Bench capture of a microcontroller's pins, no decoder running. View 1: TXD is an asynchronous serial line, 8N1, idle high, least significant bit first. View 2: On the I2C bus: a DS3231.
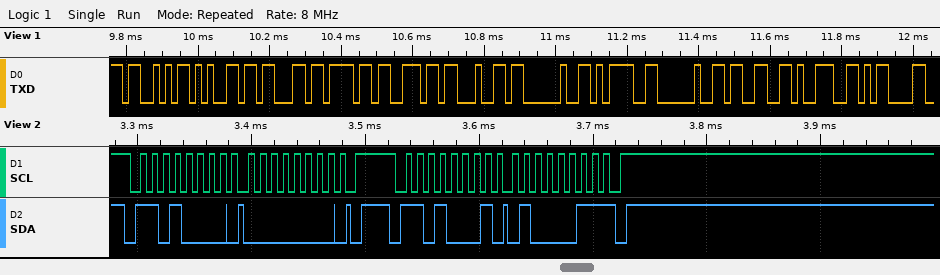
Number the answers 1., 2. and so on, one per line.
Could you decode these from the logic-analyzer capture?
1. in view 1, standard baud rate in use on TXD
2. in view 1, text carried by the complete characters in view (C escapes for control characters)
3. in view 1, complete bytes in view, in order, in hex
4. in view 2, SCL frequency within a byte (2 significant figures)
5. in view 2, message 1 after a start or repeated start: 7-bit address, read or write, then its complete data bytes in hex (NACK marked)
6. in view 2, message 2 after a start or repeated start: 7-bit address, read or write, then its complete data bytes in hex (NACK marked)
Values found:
1. 57600 baud
2. "Second = 39\r"
3. 0x53 0x65 0x63 0x6F 0x6E 0x64 0x20 0x3D 0x20 0x33 0x39 0x0D
4. 100 kHz
5. 0x68 write: 00
6. 0x68 read: 43 NACK
